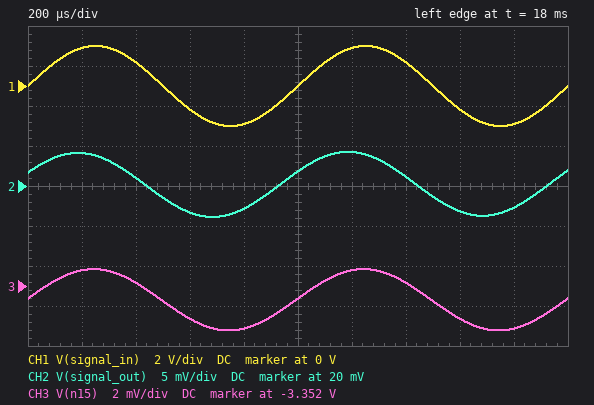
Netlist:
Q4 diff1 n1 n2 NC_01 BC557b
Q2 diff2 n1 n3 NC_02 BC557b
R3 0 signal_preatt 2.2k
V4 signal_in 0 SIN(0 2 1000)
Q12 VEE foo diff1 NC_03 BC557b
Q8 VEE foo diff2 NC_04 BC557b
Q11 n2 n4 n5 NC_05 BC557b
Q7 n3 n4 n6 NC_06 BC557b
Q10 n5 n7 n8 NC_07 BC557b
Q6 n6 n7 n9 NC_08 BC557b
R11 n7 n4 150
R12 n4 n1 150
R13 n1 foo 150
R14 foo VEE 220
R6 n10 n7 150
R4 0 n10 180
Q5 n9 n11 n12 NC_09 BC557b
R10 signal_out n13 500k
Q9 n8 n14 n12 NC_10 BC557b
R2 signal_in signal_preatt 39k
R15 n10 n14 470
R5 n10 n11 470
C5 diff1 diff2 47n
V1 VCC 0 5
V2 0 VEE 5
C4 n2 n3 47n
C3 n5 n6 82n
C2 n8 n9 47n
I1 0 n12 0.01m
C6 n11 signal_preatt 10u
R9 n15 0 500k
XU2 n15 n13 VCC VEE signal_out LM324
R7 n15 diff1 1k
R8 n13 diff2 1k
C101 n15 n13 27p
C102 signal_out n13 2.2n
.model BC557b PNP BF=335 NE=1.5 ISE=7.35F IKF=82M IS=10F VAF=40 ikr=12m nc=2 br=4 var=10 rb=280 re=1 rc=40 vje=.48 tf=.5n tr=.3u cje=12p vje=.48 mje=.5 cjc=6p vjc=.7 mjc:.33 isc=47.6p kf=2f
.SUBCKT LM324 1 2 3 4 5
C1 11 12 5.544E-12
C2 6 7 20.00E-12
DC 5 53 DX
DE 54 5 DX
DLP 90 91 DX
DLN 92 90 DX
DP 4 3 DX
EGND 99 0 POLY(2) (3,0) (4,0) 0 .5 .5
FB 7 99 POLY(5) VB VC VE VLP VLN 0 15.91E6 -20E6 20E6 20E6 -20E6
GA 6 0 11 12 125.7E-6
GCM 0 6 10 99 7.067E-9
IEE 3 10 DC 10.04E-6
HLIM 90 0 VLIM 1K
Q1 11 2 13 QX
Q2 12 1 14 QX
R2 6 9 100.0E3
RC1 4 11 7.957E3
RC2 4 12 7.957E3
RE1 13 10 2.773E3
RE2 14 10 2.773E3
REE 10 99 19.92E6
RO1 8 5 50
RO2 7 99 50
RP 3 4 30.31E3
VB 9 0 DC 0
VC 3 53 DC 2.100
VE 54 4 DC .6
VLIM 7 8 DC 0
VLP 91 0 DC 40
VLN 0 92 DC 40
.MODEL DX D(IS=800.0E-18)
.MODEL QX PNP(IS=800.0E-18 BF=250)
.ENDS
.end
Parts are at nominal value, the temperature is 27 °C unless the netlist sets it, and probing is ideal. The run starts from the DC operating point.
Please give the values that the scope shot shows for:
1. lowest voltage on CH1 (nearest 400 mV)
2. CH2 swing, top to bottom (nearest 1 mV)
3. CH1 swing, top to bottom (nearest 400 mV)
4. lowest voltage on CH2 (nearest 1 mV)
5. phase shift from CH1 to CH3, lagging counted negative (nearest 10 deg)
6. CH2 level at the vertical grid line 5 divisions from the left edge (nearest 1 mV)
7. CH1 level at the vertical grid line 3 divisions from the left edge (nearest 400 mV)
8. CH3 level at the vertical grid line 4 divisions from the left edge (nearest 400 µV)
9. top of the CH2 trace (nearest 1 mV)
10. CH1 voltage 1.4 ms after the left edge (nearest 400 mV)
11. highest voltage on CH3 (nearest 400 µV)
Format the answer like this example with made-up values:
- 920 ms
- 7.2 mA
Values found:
- -2.0 V
- 8 mV
- 4.0 V
- 16 mV
- 0 deg
- 22 mV
- -1.2 V
- -3.3540 V
- 24 mV
- 1.2 V
- -3.3512 V
